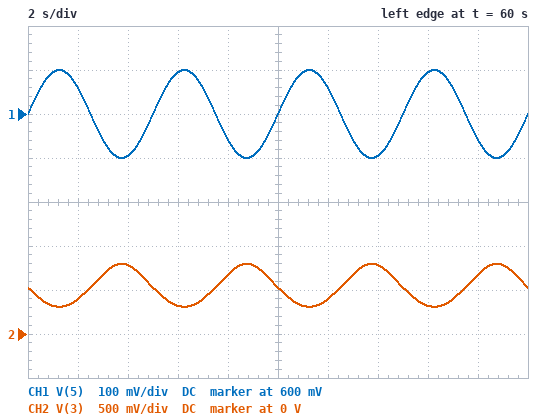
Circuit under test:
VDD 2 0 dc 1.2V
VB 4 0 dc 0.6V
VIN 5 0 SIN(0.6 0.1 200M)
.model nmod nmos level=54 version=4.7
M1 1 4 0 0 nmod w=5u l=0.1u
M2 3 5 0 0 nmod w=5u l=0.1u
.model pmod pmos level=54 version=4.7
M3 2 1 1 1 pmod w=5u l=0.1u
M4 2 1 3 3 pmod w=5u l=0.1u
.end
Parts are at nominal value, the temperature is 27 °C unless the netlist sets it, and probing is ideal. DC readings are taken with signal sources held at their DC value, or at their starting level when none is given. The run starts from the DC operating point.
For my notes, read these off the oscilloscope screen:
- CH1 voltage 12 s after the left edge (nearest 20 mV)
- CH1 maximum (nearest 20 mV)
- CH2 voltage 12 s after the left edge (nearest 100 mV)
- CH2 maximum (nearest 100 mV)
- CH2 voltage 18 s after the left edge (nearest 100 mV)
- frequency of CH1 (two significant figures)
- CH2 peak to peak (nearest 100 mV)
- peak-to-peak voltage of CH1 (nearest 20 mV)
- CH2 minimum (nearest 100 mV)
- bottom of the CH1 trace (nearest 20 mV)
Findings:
660 mV
700 mV
400 mV
800 mV
700 mV
200 mHz
500 mV
200 mV
300 mV
500 mV
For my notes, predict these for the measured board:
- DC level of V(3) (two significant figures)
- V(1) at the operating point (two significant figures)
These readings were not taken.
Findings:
530 mV
530 mV
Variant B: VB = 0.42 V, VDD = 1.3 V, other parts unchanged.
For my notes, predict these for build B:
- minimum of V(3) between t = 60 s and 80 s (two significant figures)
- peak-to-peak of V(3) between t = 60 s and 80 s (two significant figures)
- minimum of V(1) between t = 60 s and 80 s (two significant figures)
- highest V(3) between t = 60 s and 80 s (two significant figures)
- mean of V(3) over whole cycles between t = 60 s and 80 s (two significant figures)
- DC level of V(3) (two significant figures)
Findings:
110 mV
420 mV
810 mV
530 mV
260 mV
200 mV
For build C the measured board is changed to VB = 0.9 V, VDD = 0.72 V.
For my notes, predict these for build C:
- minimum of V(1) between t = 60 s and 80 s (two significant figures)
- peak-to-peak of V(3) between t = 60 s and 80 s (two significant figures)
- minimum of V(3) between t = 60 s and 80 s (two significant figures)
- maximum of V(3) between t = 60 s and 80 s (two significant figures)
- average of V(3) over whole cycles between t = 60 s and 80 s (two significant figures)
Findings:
83 mV
300 mV
140 mV
440 mV
260 mV
